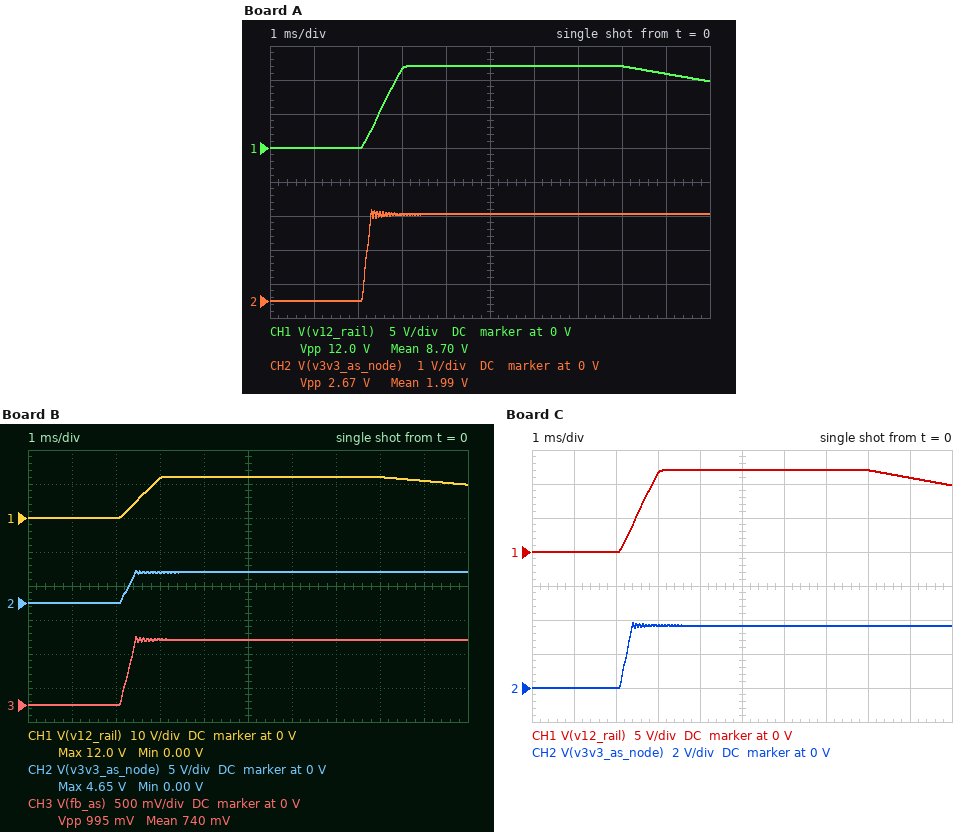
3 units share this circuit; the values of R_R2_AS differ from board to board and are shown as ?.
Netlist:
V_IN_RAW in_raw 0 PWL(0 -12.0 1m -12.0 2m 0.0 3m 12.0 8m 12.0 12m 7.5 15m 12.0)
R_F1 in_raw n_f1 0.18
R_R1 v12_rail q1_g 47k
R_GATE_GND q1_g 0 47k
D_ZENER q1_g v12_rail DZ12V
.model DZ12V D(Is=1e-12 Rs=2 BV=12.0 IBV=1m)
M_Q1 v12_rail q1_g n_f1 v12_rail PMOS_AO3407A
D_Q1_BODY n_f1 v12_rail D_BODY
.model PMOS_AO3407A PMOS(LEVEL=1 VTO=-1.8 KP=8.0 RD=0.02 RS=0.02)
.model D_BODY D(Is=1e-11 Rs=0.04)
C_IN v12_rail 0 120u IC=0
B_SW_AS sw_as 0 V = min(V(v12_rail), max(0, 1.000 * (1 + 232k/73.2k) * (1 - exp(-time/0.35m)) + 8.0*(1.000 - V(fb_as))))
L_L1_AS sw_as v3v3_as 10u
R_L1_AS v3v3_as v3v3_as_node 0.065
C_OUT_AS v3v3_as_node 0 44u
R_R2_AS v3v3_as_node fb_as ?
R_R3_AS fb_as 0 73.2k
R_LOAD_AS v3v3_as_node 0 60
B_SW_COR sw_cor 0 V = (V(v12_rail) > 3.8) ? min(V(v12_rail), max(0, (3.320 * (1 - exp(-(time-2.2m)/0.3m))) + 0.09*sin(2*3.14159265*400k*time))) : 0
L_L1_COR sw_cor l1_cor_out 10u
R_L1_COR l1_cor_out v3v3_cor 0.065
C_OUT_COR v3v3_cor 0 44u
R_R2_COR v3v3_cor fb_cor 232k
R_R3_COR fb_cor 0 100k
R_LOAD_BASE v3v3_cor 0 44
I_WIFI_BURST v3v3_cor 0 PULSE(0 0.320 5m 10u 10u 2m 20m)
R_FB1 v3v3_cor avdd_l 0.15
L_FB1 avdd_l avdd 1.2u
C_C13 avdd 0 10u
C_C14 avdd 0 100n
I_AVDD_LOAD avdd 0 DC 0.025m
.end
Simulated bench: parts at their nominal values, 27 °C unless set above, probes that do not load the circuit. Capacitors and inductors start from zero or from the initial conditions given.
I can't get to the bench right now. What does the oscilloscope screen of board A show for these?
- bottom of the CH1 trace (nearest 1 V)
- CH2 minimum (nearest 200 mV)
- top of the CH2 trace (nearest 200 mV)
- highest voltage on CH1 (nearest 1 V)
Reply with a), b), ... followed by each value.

a) 0 V
b) 0 V
c) 2.6 V
d) 12 V
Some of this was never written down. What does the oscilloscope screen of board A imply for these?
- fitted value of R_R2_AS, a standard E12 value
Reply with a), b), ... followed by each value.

a) 82 kΩ
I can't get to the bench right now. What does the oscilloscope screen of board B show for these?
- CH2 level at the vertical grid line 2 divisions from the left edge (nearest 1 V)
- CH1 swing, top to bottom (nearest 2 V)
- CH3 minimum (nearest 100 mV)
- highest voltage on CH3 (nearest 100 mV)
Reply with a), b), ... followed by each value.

a) 0 V
b) 12 V
c) 0 V
d) 1.0 V
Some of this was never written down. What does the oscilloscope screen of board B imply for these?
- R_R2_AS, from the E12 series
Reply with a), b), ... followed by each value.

a) 270 kΩ
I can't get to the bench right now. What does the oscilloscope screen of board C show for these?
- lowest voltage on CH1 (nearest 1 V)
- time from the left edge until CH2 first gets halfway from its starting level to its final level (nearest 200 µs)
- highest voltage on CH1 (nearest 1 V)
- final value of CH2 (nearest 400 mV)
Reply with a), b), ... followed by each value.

a) 0 V
b) 2.2 ms
c) 12 V
d) 3.6 V
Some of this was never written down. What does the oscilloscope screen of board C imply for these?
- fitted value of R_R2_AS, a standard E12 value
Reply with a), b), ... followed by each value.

a) 180 kΩ
